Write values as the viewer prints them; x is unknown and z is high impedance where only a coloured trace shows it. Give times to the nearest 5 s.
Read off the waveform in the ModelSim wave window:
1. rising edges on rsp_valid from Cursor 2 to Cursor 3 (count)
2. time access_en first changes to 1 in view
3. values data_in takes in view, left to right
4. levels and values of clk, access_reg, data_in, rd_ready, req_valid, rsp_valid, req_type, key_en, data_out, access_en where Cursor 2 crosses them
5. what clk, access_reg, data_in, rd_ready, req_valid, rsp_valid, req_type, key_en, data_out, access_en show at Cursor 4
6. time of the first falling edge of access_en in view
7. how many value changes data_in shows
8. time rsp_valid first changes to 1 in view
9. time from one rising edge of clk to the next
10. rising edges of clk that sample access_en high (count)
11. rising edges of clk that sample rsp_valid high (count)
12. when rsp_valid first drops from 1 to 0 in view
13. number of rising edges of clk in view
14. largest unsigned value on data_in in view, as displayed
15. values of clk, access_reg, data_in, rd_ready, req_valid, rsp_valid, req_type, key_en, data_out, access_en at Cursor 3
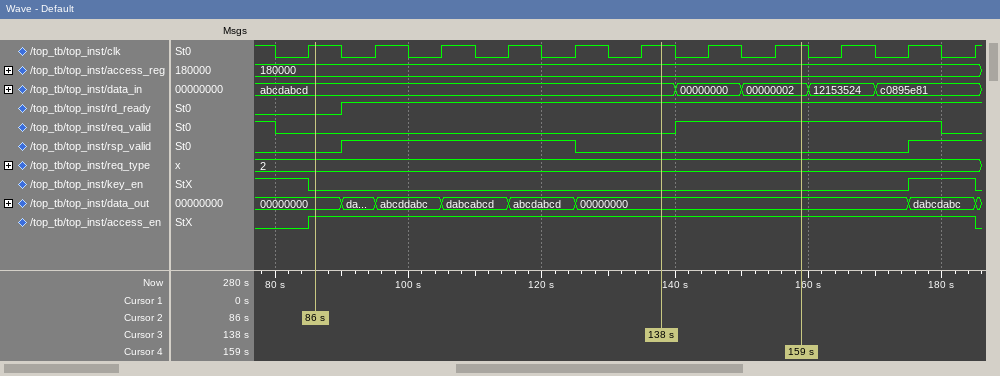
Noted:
1
85 s
abcdabcd, 00000000, 00000002, 12153524, c0895e81
clk=1, access_reg=180000, data_in=abcdabcd, rd_ready=0, req_valid=0, rsp_valid=0, req_type=2, key_en=0, data_out=00000000, access_en=1
clk=1, access_reg=180000, data_in=00000002, rd_ready=1, req_valid=1, rsp_valid=0, req_type=2, key_en=0, data_out=00000000, access_en=1
185 s
4
90 s
10 s
10
5
125 s
11
c0895e81
clk=1, access_reg=180000, data_in=abcdabcd, rd_ready=1, req_valid=0, rsp_valid=0, req_type=2, key_en=0, data_out=00000000, access_en=1
